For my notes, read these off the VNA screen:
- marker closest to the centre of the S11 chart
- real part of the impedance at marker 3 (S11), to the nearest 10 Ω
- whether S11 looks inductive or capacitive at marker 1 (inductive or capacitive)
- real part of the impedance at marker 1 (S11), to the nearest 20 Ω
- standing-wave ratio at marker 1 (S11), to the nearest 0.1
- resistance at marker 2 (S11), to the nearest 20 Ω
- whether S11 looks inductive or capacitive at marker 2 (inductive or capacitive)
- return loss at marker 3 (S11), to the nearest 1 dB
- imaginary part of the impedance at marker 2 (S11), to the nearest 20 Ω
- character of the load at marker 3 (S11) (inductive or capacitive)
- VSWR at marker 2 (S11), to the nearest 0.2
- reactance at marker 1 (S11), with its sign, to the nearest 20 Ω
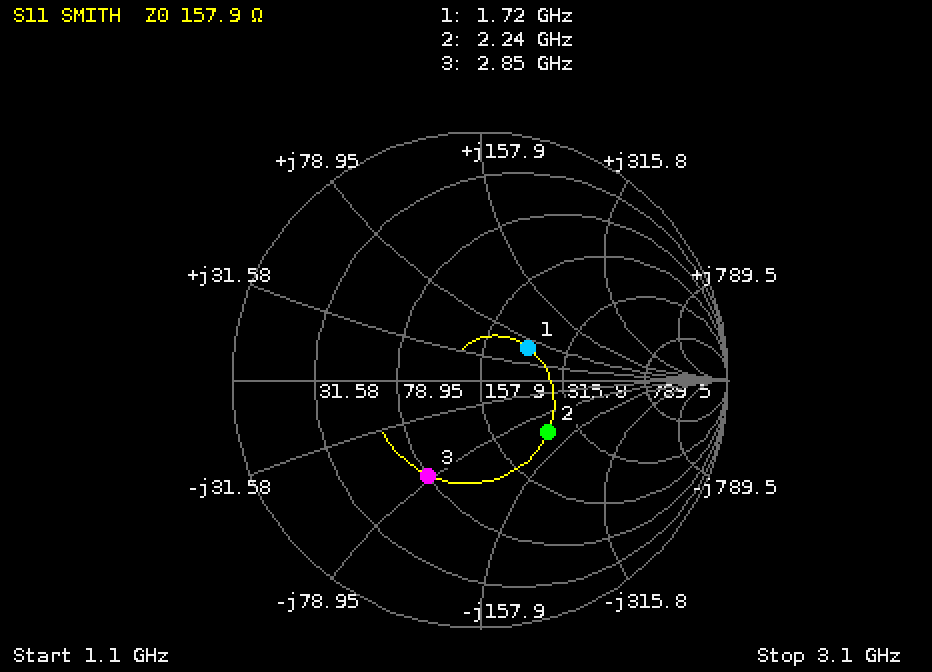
marker 1
80 Ω
inductive
220 Ω
1.6
240 Ω
capacitive
7 dB
-120 Ω
capacitive
2.0
+60 Ω
